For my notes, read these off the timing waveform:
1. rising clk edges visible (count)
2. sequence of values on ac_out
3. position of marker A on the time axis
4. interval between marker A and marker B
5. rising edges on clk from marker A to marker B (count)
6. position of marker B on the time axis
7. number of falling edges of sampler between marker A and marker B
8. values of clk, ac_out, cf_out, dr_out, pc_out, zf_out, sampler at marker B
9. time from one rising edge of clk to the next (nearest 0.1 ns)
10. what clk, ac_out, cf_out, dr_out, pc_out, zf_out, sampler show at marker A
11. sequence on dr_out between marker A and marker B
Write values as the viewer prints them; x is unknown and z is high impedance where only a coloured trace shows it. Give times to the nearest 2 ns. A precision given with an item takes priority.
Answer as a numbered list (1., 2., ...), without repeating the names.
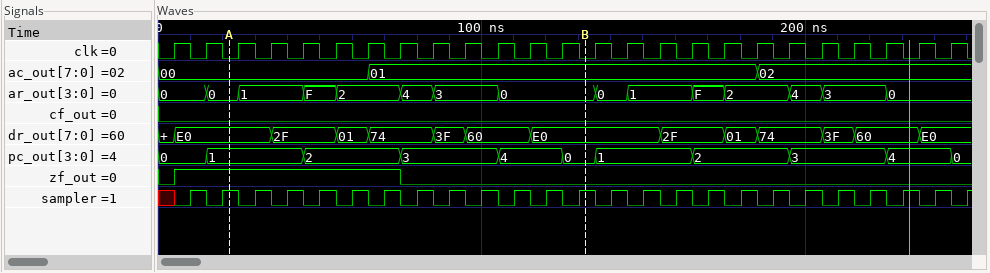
1. 25
2. 00, 01, 02
3. 22 ns
4. 110 ns
5. 11
6. 132 ns
7. 11
8. clk=0, ac_out=01, cf_out=0, dr_out=E0, pc_out=0, zf_out=0, sampler=1
9. 10 ns
10. clk=0, ac_out=00, cf_out=0, dr_out=E0, pc_out=1, zf_out=1, sampler=1
11. E0, 2F, 01, 74, 3F, 60, E0
